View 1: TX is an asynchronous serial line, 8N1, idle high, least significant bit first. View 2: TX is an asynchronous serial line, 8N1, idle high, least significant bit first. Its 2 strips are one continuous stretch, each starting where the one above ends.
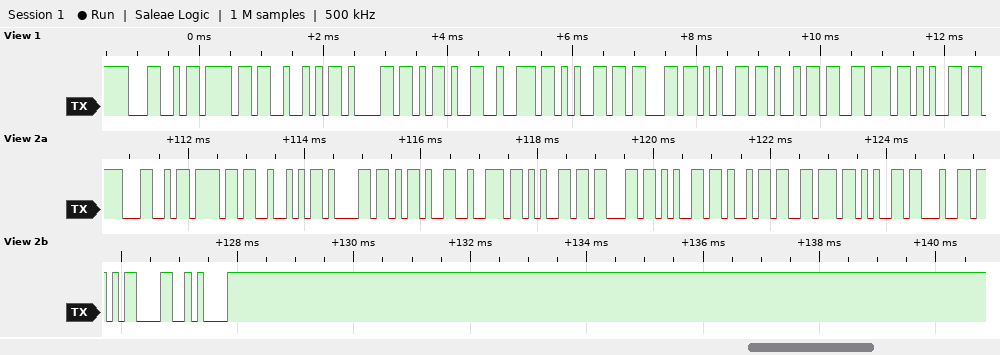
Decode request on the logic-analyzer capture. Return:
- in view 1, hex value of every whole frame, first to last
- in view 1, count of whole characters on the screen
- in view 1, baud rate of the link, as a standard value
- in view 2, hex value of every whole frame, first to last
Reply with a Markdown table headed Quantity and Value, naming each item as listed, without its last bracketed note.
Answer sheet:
| Quantity | Value |
|---|---|
| in view 1, hex value of every whole frame, first to last | 4C 6F 52 61 2D 72 65 63 65 69 76 65 |
| in view 1, count of whole characters on the screen | 12 |
| in view 1, baud rate of the link, as a standard value | 9600 baud |
| in view 2, hex value of every whole frame, first to last | 4C 6F 52 61 2D 72 65 63 65 69 76 65 64 0D 0A |
